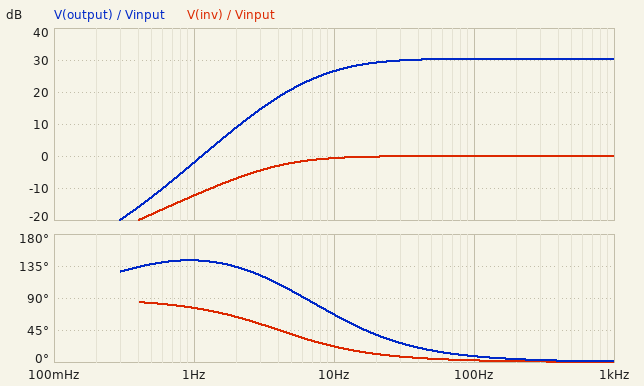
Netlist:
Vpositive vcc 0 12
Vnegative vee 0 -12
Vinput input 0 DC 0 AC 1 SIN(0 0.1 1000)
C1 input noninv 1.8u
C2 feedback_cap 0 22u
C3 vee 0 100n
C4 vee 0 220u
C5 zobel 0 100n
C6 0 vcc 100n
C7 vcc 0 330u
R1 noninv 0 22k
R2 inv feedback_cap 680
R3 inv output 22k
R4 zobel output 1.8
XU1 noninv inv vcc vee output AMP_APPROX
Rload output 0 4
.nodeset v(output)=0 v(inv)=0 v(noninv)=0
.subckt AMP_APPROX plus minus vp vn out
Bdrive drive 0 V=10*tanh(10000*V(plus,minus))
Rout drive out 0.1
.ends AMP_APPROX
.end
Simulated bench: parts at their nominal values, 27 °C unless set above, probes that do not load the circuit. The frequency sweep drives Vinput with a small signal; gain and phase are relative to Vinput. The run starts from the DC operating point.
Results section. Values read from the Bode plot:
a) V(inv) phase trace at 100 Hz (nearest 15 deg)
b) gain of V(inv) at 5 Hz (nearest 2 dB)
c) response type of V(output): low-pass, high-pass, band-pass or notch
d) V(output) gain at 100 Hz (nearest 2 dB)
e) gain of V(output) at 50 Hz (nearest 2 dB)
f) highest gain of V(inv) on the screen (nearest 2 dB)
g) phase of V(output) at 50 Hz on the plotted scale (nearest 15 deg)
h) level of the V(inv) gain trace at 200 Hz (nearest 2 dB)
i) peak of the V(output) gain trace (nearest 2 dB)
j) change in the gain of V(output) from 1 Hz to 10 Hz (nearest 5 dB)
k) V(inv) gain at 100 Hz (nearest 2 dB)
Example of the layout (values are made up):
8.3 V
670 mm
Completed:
0 deg
-2 dB
high-pass
30 dB
30 dB
0 dB
15 deg
0 dB
30 dB
30 dB
0 dB
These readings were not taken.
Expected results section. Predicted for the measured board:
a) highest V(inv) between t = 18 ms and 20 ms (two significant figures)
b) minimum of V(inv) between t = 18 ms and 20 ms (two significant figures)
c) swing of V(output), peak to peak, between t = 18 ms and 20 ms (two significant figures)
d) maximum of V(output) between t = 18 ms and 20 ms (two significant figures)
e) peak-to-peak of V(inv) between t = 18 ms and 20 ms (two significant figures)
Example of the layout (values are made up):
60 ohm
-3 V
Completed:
100 mV
-100 mV
6.7 V
3.3 V
200 mV
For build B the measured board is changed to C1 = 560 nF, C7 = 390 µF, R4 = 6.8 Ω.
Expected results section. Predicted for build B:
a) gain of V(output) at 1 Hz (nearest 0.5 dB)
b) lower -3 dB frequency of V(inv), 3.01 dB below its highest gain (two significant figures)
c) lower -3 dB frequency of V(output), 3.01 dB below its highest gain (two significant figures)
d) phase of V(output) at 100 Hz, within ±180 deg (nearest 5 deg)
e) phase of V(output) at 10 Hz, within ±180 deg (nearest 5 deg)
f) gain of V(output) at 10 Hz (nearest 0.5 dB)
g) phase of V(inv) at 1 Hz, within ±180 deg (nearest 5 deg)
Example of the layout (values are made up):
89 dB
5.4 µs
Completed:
-12.0 dB
13 Hz
18 Hz
15 deg
95 deg
23.0 dB
85 deg
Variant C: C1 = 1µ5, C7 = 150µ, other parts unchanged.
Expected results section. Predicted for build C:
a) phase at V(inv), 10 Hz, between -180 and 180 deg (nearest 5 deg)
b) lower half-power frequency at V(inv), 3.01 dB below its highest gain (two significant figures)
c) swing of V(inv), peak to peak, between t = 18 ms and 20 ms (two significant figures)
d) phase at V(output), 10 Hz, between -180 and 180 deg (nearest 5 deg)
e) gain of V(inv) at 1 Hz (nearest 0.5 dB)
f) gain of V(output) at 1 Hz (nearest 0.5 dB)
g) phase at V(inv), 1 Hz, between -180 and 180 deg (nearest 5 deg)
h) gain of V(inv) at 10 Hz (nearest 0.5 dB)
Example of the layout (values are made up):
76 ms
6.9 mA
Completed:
25 deg
4.8 Hz
200 mV
70 deg
-14.0 dB
-3.5 dB
80 deg
-1.0 dB
